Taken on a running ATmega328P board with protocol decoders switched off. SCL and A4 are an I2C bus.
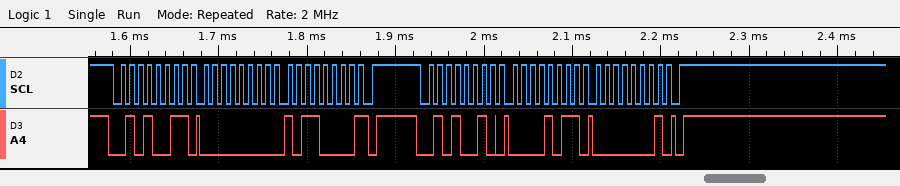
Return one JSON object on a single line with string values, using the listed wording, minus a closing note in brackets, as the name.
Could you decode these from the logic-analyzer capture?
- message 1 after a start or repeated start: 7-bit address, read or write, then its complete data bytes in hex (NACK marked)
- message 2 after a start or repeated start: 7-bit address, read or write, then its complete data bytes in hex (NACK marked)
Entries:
{"message 1 after a start or repeated start: 7-bit address, read or write, then its complete data bytes in hex": "0x29 read: 00 B0 NACK", "message 2 after a start or repeated start: 7-bit address, read or write, then its complete data bytes in hex": "0x29 write: 0B 01"}
